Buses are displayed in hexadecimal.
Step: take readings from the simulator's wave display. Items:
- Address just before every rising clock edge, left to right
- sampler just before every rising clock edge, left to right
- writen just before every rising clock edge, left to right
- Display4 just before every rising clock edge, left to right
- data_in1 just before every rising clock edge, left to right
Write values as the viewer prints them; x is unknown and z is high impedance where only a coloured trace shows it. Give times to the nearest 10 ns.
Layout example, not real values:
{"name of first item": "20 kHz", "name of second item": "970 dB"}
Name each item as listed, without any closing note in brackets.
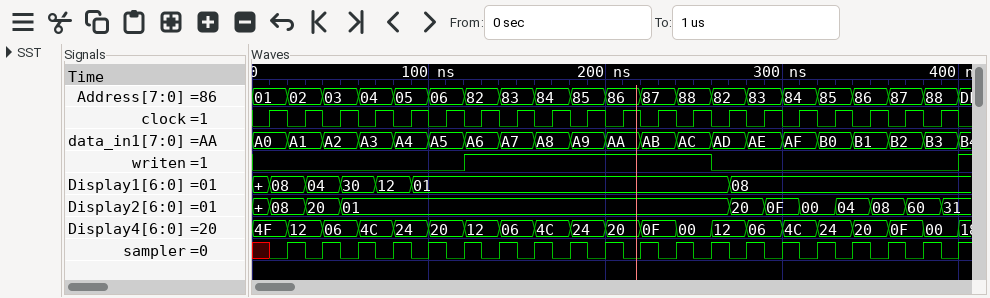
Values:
{"Address just before every rising clock edge, left to right": "01, 02, 03, 04, 05, 06, 82, 83, 84, 85, 86, 87, 88, 82, 83, 84, 85, 86, 87, 88", "sampler just before every rising clock edge, left to right": "x 1 1 1 1 1 1 1 1 1 1 1 1 1 1 1 1 1 1 1", "writen just before every rising clock edge, left to right": "0 0 0 0 0 0 1 1 1 1 1 1 1 0 0 0 0 0 0 0", "Display4 just before every rising clock edge, left to right": "4F, 12, 06, 4C, 24, 20, 12, 06, 4C, 24, 20, 0F, 00, 12, 06, 4C, 24, 20, 0F, 00", "data_in1 just before every rising clock edge, left to right": "A0, A1, A2, A3, A4, A5, A6, A7, A8, A9, AA, AB, AC, AD, AE, AF, B0, B1, B2, B3"}
